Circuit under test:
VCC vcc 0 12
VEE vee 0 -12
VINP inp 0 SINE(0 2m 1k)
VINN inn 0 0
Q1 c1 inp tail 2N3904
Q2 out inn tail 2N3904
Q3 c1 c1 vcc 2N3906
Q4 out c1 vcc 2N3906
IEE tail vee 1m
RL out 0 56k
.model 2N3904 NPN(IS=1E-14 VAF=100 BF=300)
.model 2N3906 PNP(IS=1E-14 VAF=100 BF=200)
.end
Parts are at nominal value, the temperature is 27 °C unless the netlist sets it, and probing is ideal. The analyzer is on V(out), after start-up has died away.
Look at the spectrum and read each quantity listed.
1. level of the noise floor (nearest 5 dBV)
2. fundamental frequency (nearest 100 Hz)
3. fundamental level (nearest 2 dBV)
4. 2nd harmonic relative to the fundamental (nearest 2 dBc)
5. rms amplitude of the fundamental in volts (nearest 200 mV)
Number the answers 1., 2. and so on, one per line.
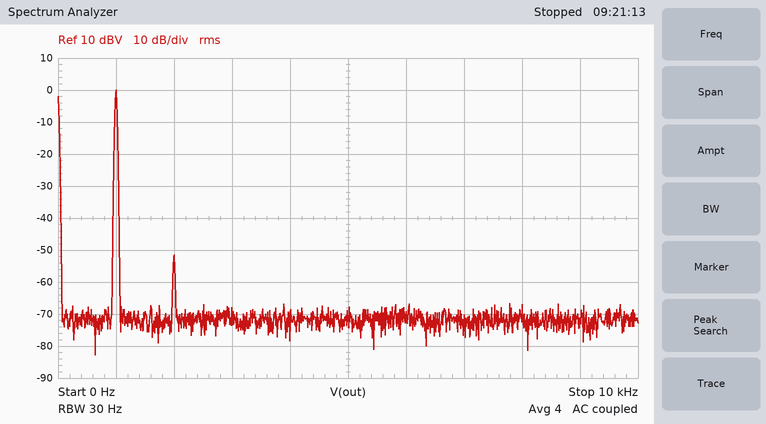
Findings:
1. -70 dBV
2. 1.0 kHz
3. 0 dBV
4. -52 dBc
5. 1.0 V
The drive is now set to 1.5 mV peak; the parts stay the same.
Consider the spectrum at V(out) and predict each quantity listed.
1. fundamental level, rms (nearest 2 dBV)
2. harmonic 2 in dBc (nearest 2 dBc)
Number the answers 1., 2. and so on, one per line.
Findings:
1. -2 dBV
2. -54 dBc
